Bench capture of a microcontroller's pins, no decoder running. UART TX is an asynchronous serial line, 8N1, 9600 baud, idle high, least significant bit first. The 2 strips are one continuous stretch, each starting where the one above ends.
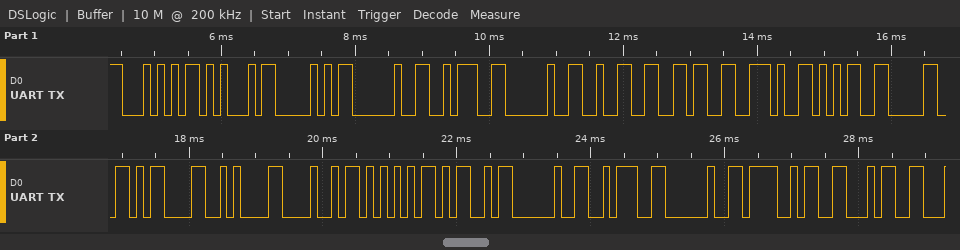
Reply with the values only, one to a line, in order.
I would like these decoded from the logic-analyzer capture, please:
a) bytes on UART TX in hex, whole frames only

54 45 50 20 3A 20 32 36 2E 35 30 0D 0A 48 55 4D 20 3A 20 4F 46
